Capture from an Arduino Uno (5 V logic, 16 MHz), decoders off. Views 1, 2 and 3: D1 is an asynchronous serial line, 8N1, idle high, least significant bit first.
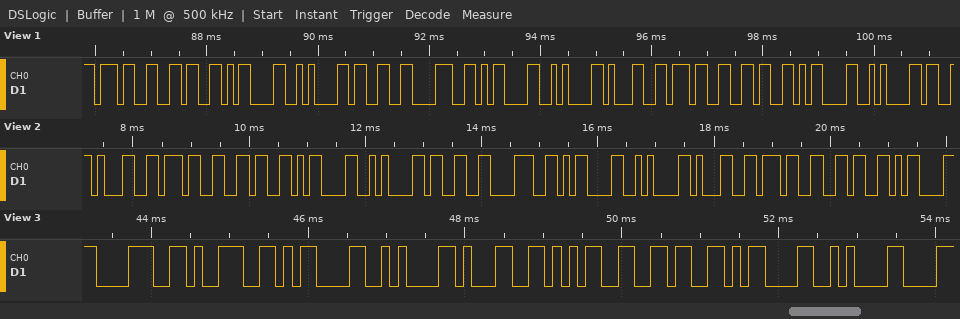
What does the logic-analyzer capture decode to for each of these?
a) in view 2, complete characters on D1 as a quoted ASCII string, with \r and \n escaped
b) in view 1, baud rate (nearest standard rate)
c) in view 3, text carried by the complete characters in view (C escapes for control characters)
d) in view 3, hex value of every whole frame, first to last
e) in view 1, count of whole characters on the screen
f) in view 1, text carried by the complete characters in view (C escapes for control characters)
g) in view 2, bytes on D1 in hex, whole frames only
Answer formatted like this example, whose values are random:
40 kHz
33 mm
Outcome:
"176\r\n38\r\n176\r"
9600 baud
"89\r\n156\r\n"
0x38 0x39 0x0D 0x0A 0x31 0x35 0x36 0x0D 0x0A
13
"76\r\n38\r\n176\r\n"
0x31 0x37 0x36 0x0D 0x0A 0x33 0x38 0x0D 0x0A 0x31 0x37 0x36 0x0D
